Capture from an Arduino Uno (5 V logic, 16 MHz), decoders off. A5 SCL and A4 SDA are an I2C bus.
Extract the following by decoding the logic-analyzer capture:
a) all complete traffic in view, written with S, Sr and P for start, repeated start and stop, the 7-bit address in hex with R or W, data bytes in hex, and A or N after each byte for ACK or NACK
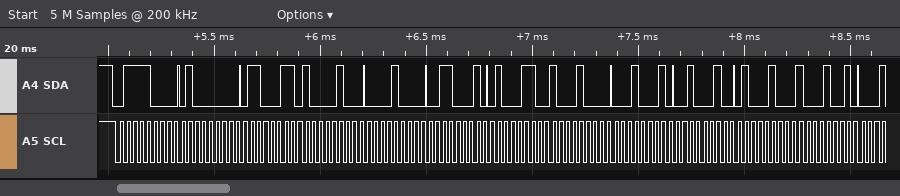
S 3CW A 40 A 63 A 84 A 08 A 31 A 46 A 88 A 11 A 22 A 44 A 89 A
